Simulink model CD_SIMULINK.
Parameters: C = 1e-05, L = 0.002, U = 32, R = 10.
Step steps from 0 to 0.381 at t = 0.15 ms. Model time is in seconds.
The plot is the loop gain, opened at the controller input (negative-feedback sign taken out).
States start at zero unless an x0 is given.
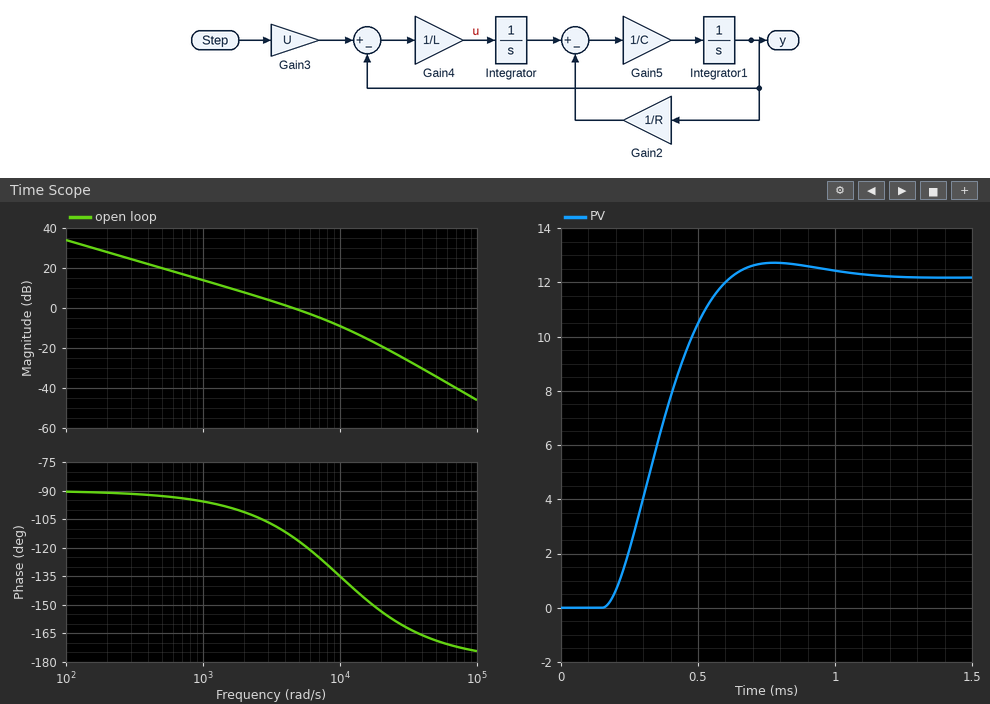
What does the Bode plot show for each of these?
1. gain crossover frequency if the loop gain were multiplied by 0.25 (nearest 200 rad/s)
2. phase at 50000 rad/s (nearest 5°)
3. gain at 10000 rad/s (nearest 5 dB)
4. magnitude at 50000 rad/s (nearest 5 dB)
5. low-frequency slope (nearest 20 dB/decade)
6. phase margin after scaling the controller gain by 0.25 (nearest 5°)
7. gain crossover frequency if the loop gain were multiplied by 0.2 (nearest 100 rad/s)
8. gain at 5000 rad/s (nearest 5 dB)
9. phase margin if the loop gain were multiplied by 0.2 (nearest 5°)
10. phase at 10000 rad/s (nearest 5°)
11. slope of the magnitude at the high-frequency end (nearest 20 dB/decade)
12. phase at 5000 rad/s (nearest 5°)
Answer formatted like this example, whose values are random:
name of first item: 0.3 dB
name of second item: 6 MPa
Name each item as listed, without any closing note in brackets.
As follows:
gain crossover frequency if the loop gain were multiplied by 0.25: 1200 rad/s
phase at 50000 rad/s: -170°
gain at 10000 rad/s: -10 dB
magnitude at 50000 rad/s: -35 dB
low-frequency slope: -20 dB/decade
phase margin after scaling the controller gain by 0.25: 85°
gain crossover frequency if the loop gain were multiplied by 0.2: 1000 rad/s
gain at 5000 rad/s: 0 dB
phase margin if the loop gain were multiplied by 0.2: 85°
phase at 10000 rad/s: -135°
slope of the magnitude at the high-frequency end: -40 dB/decade
phase at 5000 rad/s: -115°
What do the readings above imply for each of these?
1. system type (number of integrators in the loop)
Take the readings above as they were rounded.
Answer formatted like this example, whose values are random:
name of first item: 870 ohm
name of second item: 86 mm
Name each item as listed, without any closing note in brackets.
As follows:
system type: 1
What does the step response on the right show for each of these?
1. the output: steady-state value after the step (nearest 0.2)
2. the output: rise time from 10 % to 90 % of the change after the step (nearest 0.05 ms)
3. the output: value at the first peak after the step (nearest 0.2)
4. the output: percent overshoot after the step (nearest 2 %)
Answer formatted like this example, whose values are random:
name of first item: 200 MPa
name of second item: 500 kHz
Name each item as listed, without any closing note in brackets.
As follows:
the output: steady-state value after the step: 12.2
the output: rise time from 10 % to 90 % of the change after the step: 0.30 ms
the output: value at the first peak after the step: 12.8
the output: percent overshoot after the step: 4 %
